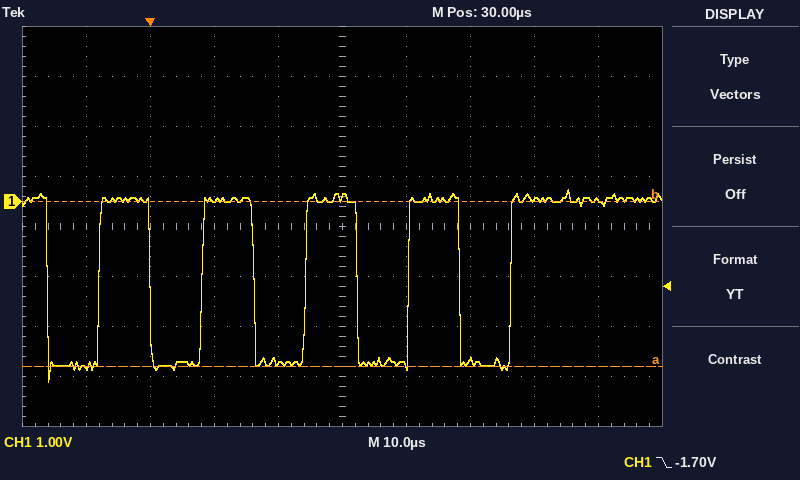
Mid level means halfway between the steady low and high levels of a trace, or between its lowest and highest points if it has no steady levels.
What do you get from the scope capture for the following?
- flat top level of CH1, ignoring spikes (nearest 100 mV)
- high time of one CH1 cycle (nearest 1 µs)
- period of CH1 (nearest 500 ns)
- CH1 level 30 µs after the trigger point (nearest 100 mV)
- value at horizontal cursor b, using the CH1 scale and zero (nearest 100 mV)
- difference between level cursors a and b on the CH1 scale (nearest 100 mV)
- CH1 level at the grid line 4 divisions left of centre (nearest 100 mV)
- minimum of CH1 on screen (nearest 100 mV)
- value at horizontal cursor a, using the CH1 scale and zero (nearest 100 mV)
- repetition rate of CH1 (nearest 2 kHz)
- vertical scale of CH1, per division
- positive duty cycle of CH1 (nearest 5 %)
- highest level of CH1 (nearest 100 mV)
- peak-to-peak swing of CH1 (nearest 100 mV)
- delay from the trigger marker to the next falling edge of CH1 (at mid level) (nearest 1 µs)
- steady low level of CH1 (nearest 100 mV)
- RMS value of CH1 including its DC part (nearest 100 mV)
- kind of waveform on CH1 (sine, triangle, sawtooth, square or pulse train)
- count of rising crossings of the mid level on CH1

0.0 V
8 µs
16.0 µs
100 mV
0.0 V
3.3 V
-3.3 V
-3.6 V
-3.3 V
62 kHz
1 V
50 %
200 mV
3.8 V
16 µs
-3.3 V
2.3 V
square
5
